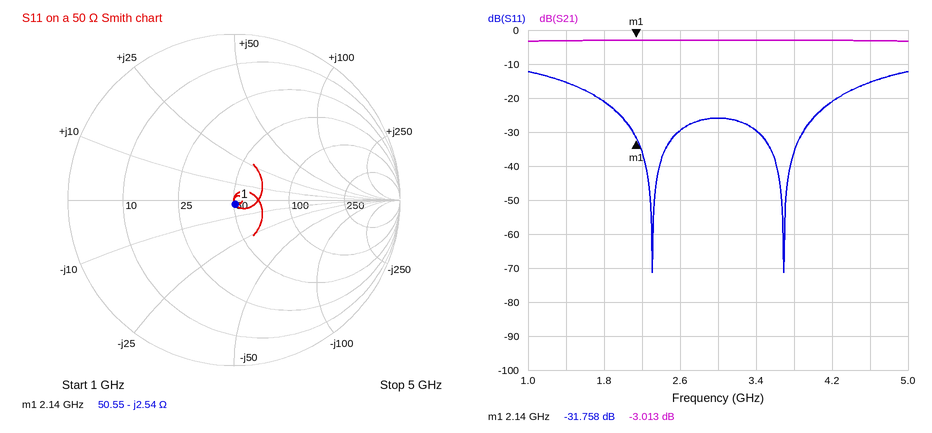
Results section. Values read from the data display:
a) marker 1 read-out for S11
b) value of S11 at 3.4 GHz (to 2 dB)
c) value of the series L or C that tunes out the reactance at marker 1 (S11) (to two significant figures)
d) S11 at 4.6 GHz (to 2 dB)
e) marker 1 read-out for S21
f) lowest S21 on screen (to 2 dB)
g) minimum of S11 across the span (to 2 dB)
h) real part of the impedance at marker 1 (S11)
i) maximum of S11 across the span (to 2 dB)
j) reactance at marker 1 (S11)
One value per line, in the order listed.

-31.758 dB
-30 dB
190 pH
-16 dB
-3.013 dB
-4 dB
-72 dB
50.55 Ω
-12 dB
-2.54 Ω
